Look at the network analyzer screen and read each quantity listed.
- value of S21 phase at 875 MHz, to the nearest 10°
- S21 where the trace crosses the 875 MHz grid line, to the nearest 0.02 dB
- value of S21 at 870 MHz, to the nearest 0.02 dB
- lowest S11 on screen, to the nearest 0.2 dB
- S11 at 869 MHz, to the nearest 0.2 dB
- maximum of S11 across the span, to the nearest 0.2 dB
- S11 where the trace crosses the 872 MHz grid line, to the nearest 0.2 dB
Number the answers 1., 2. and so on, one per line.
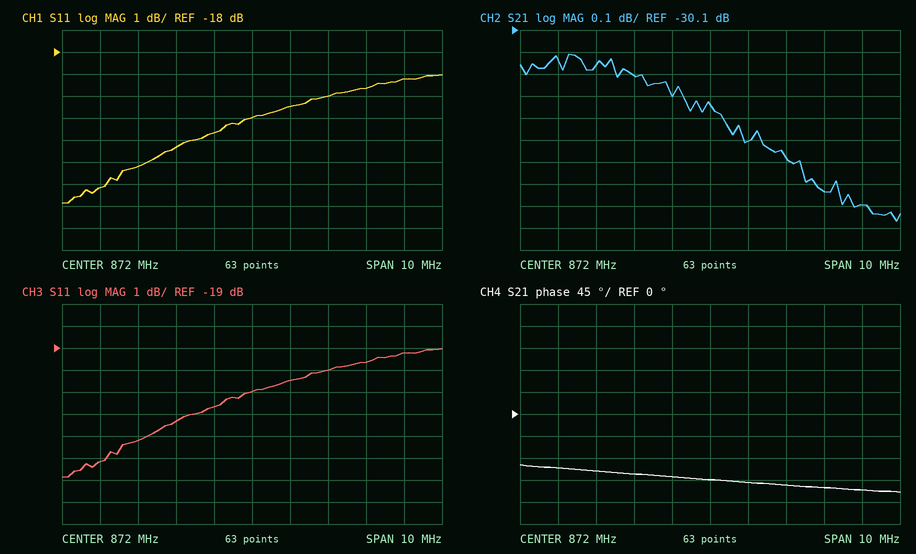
1. -150°
2. -30.84 dB
3. -30.30 dB
4. -24.8 dB
5. -23.2 dB
6. -19.0 dB
7. -21.0 dB
